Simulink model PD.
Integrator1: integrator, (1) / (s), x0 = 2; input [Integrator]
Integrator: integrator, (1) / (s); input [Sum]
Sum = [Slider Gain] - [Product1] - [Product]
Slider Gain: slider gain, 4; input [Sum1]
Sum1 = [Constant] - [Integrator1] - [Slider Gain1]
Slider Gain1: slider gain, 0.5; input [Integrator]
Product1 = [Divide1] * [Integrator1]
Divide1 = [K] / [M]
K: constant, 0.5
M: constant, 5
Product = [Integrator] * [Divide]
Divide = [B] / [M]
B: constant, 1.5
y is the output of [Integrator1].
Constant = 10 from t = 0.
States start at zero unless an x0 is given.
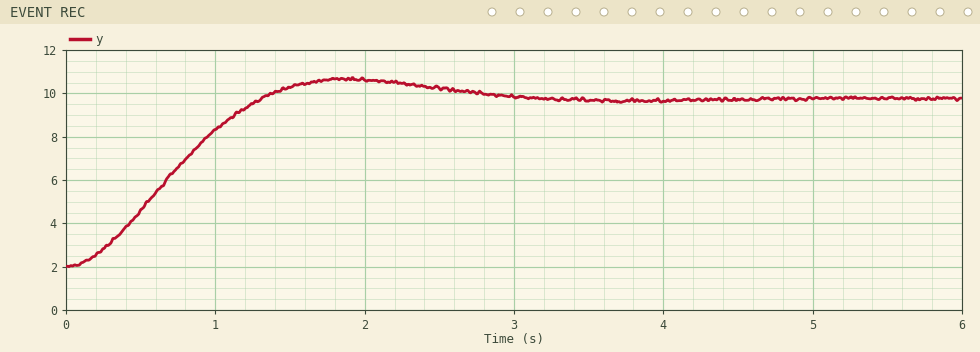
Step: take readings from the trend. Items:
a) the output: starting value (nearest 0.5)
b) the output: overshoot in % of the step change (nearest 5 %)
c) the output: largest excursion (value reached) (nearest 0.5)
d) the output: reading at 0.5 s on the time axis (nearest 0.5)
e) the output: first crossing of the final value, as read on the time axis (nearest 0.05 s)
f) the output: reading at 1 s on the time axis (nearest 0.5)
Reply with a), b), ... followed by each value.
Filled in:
a) 2.0
b) 10 %
c) 10.5
d) 4.5
e) 1.30 s
f) 8.5
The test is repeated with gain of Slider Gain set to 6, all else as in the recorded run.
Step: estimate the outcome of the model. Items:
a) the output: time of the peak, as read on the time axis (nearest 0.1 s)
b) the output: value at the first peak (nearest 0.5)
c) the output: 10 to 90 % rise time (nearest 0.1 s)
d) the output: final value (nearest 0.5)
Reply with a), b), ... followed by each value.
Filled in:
a) 1.7 s
b) 10.5
c) 0.8 s
d) 10.0
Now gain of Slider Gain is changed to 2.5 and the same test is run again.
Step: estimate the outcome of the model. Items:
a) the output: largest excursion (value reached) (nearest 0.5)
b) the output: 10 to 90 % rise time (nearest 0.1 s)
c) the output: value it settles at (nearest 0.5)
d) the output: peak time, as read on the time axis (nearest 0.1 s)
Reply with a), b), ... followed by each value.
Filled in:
a) 11.0
b) 1.0 s
c) 9.5
d) 2.2 s
